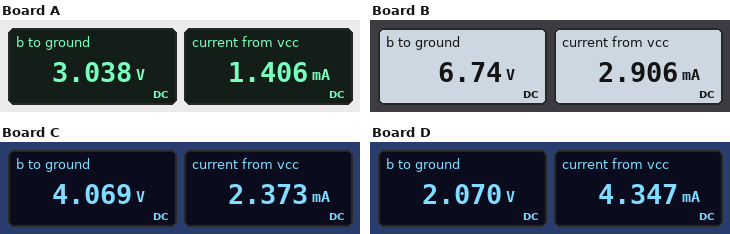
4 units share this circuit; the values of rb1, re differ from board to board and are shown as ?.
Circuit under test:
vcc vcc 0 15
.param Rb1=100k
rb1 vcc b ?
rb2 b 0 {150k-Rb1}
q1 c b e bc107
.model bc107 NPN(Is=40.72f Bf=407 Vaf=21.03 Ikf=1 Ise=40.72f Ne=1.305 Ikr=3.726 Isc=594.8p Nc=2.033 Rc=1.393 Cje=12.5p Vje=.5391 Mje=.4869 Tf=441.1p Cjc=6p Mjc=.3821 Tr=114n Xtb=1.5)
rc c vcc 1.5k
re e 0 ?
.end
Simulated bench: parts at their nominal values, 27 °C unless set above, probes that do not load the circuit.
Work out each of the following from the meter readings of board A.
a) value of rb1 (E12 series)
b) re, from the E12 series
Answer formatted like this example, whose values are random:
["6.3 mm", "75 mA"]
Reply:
["180 kΩ", "1.8 kΩ"]
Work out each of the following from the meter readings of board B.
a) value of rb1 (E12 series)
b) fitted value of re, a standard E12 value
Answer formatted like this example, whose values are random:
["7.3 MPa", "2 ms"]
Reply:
["56 kΩ", "2.2 kΩ"]
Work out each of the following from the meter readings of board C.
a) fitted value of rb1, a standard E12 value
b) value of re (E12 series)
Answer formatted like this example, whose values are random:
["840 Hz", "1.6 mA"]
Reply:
["120 kΩ", "1.5 kΩ"]
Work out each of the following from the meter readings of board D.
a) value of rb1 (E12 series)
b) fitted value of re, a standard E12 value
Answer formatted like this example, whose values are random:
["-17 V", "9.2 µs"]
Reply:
["220 kΩ", "330 Ω"]
